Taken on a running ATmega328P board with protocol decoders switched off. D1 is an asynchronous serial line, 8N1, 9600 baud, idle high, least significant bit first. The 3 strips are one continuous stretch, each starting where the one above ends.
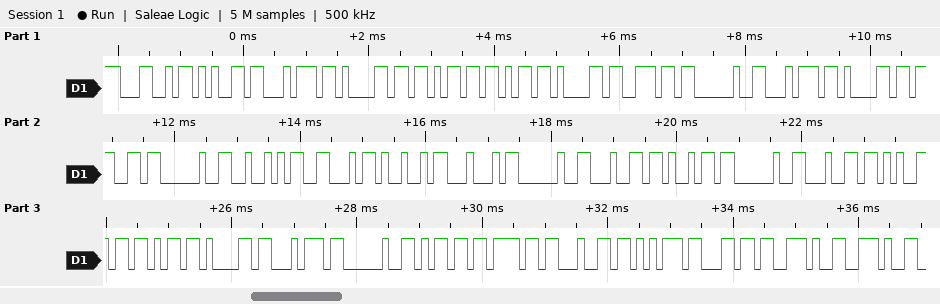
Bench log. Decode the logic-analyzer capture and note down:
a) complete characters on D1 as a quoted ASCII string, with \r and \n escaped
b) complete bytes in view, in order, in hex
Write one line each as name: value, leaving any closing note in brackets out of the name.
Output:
complete characters on D1 as a quoted ASCII string, with \r and \n escaped: "Letakkan tag RFID di dekat modul.."
complete bytes in view, in order, in hex: 4C 65 74 61 6B 6B 61 6E 20 74 61 67 20 52 46 49 44 20 64 69 20 64 65 6B 61 74 20 6D 6F 64 75 6C 2E 2E
